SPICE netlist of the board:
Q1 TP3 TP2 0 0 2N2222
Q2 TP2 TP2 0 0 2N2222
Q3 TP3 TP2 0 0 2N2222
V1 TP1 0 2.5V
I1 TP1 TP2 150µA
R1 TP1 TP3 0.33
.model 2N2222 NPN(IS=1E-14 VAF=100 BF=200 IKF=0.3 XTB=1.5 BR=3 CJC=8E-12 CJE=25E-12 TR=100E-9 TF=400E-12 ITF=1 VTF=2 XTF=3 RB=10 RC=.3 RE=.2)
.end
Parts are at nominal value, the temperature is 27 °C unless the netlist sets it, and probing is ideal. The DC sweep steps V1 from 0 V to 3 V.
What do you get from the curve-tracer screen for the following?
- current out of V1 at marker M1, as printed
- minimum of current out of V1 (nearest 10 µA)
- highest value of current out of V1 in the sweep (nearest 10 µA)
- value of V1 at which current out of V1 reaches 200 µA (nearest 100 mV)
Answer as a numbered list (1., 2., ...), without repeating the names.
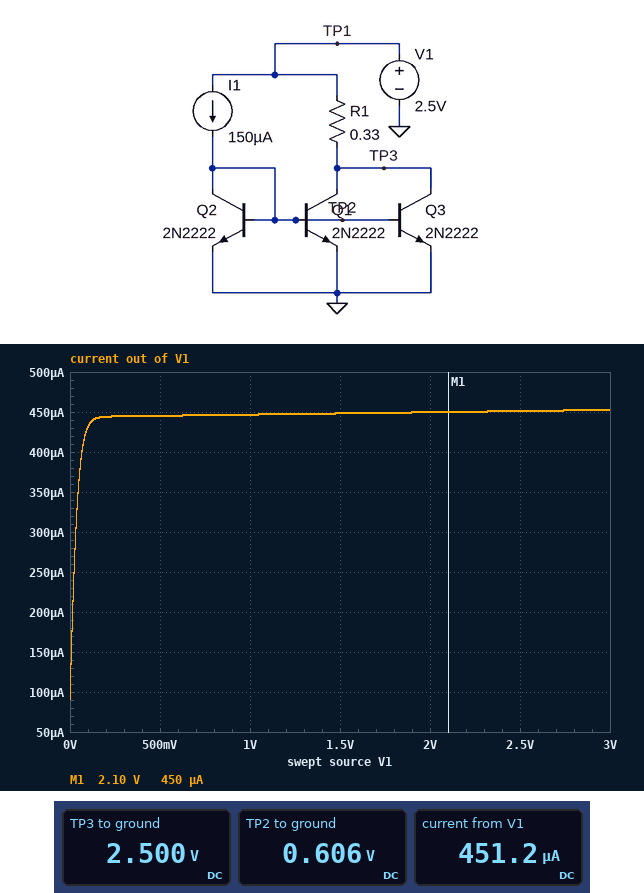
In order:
1. 450 µA
2. 90 µA
3. 450 µA
4. 0 V
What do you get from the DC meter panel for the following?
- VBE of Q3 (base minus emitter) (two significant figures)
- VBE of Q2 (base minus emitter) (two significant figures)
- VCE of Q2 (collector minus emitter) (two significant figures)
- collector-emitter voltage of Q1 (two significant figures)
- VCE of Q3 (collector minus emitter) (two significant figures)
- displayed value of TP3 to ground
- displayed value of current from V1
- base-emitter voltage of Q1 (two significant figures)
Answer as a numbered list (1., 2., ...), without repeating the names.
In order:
1. 610 mV
2. 610 mV
3. 610 mV
4. 2.5 V
5. 2.5 V
6. 2.500 V
7. 451.2 µA
8. 610 mV
